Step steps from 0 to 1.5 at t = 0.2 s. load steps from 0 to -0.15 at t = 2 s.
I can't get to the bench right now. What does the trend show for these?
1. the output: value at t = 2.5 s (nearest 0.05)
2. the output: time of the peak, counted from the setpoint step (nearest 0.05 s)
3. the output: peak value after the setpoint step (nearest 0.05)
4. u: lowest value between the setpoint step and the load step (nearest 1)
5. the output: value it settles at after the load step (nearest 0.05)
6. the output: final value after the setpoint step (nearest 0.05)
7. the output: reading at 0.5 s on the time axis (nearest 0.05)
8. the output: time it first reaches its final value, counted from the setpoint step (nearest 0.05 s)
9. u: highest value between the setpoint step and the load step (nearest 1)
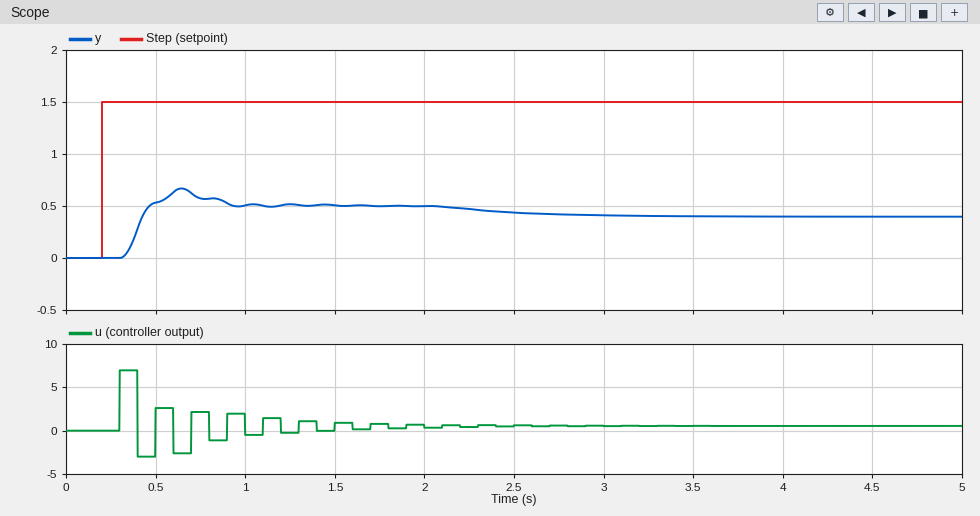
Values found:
0.45
0.45 s
0.65
-3
0.40
0.50
0.55
0.25 s
7
